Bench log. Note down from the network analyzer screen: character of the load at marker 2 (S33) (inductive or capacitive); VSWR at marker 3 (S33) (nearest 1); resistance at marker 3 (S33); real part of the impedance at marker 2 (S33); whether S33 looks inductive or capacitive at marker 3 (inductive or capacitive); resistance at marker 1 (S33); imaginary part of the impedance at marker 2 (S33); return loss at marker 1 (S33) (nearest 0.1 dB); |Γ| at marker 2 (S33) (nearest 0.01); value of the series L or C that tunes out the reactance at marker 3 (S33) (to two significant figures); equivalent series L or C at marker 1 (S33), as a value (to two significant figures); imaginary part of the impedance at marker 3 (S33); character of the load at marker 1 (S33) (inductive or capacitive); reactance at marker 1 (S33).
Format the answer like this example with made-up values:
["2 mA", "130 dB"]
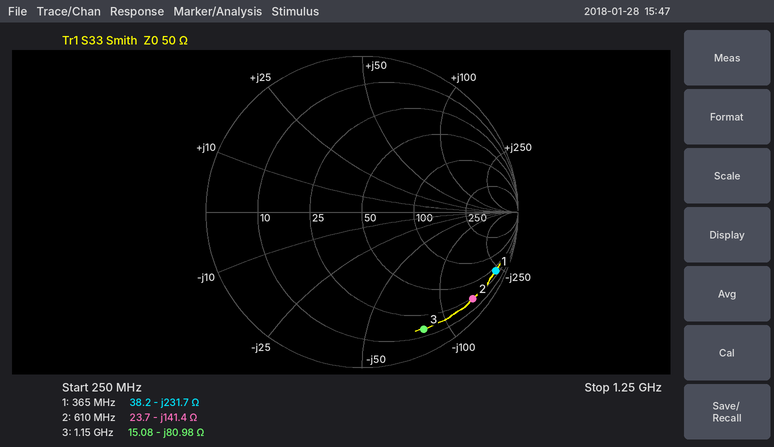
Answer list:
["capacitive", "12", "15.08 Ω", "23.7 Ω", "capacitive", "38.2 Ω", "-141.4 Ω", "0.6 dB", "0.90", "11 nH", "1.9 pF", "-80.98 Ω", "capacitive", "-231.7 Ω"]
